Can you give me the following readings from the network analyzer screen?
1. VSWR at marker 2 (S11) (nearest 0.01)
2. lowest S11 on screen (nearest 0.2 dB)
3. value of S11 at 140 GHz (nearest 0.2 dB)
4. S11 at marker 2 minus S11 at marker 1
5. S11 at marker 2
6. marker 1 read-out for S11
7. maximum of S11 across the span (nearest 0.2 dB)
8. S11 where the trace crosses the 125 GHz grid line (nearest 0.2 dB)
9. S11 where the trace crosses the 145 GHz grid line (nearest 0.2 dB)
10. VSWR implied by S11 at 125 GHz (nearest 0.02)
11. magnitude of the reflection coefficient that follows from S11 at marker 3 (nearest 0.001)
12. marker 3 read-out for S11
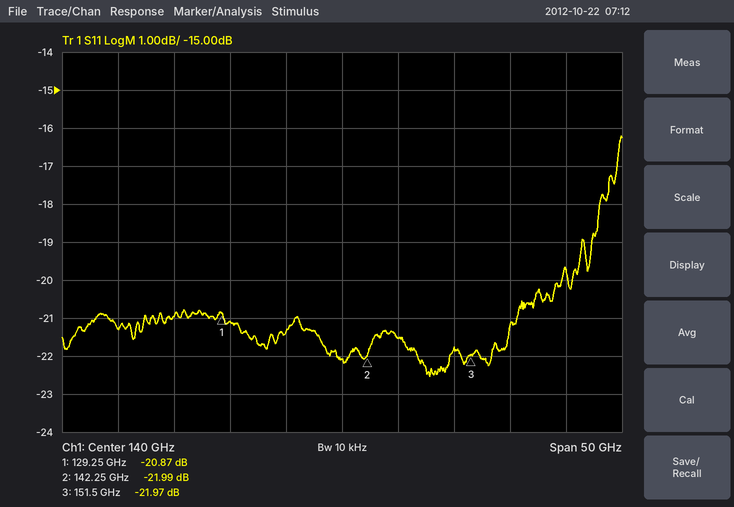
1.17
-22.6 dB
-22.0 dB
-1.12 dB
-21.99 dB
-20.87 dB
-16.2 dB
-21.0 dB
-21.6 dB
1.20
0.080
-21.97 dB
